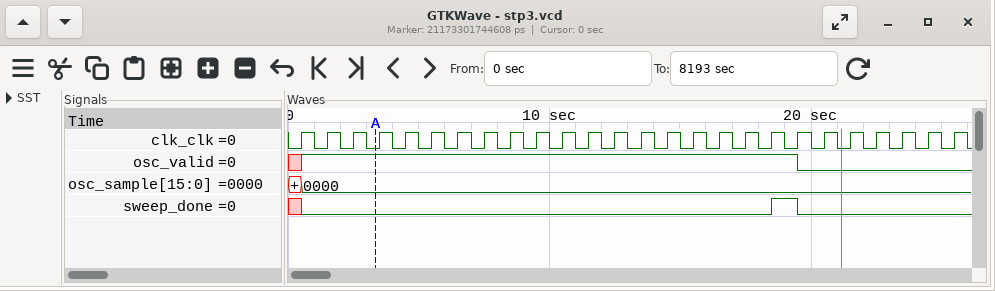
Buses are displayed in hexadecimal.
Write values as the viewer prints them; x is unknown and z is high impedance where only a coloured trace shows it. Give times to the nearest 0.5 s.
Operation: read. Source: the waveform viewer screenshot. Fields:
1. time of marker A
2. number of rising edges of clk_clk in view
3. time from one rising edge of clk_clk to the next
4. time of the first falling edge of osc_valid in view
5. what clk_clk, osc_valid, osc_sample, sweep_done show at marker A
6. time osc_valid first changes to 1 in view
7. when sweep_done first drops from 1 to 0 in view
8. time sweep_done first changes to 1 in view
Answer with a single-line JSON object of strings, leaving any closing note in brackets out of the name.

{"time of marker A": "3.5 s", "number of rising edges of clk_clk in view": "26", "time from one rising edge of clk_clk to the next": "1 s", "time of the first falling edge of osc_valid in view": "19.5 s", "what clk_clk, osc_valid, osc_sample, sweep_done show at marker A": "clk_clk=0, osc_valid=1, osc_sample=0000, sweep_done=0", "time osc_valid first changes to 1 in view": "0.5 s", "when sweep_done first drops from 1 to 0 in view": "19.5 s", "time sweep_done first changes to 1 in view": "18.5 s"}
